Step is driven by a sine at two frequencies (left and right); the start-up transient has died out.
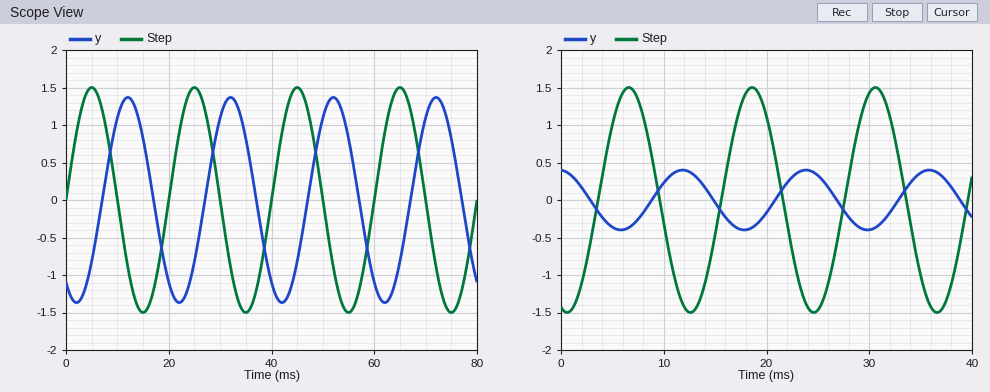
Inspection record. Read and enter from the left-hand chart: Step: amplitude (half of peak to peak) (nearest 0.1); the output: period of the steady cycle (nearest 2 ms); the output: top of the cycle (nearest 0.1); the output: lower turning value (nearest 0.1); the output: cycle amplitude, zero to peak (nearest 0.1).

1.5
20 ms
1.4
-1.4
1.4
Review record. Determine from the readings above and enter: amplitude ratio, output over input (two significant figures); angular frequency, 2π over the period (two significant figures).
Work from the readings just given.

0.93
0.31 rad/ms
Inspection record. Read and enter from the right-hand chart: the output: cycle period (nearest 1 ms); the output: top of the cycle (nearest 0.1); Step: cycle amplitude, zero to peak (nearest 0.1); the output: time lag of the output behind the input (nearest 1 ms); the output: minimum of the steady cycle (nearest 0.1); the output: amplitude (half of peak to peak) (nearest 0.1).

12 ms
0.4
1.5
5 ms
-0.4
0.4
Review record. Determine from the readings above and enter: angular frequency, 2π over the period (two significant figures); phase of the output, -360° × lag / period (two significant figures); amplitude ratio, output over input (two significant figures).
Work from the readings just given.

0.52 rad/ms
-150°
0.27
